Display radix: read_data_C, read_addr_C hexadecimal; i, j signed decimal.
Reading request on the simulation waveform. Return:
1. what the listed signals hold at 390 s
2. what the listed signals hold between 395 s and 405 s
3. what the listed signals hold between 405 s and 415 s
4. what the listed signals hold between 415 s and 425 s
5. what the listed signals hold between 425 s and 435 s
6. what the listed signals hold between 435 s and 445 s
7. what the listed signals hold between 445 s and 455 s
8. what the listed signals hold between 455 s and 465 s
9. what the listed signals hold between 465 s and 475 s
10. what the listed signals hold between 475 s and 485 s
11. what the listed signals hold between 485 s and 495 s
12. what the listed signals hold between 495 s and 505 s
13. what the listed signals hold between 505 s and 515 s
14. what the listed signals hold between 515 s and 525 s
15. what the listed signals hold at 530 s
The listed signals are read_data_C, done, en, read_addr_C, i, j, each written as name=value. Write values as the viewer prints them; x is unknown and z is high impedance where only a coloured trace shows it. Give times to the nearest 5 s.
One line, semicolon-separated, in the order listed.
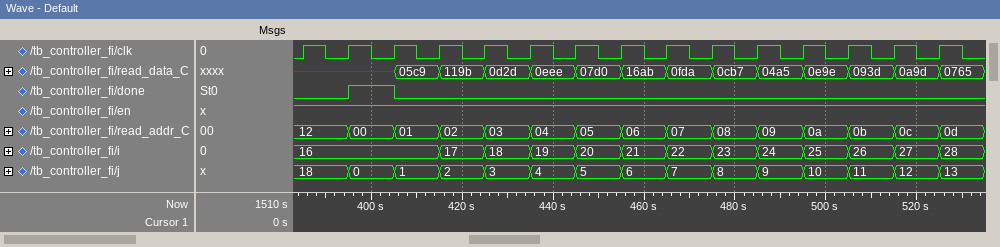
read_data_C=x, done=0, en=1, read_addr_C=12, i=16, j=18; read_data_C=x, done=1, en=1, read_addr_C=00, i=16, j=0; read_data_C=05c9, done=0, en=1, read_addr_C=01, i=16, j=1; read_data_C=119b, done=0, en=1, read_addr_C=02, i=17, j=2; read_data_C=0d2d, done=0, en=1, read_addr_C=03, i=18, j=3; read_data_C=0eee, done=0, en=1, read_addr_C=04, i=19, j=4; read_data_C=07d0, done=0, en=1, read_addr_C=05, i=20, j=5; read_data_C=16ab, done=0, en=1, read_addr_C=06, i=21, j=6; read_data_C=0fda, done=0, en=1, read_addr_C=07, i=22, j=7; read_data_C=0cb7, done=0, en=1, read_addr_C=08, i=23, j=8; read_data_C=04a5, done=0, en=1, read_addr_C=09, i=24, j=9; read_data_C=0e9e, done=0, en=1, read_addr_C=0a, i=25, j=10; read_data_C=093d, done=0, en=1, read_addr_C=0b, i=26, j=11; read_data_C=0a9d, done=0, en=1, read_addr_C=0c, i=27, j=12; read_data_C=0765, done=0, en=1, read_addr_C=0d, i=28, j=13
